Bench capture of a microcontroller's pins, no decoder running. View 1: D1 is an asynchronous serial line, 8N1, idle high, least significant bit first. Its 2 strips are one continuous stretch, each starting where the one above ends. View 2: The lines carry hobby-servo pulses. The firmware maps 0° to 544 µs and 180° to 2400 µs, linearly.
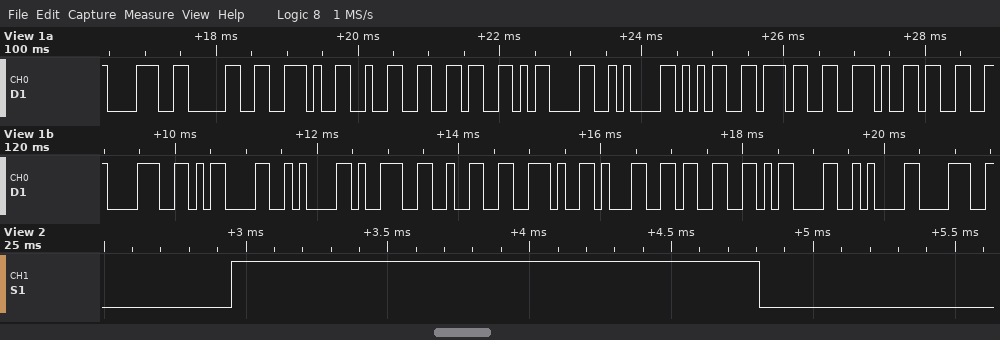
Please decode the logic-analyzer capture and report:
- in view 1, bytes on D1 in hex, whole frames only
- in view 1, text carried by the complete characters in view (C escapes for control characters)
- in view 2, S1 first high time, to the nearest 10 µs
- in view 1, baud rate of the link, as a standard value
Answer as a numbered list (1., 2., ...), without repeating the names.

1. 38 30 2E 32 36 0D 0A 35 37 2E 33 38 0D 0A 39 32 2E 31 33 0D 0A 38
2. "80.26\r\n57.38\r\n92.13\r\n8"
3. 1860 µs
4. 9600 baud
